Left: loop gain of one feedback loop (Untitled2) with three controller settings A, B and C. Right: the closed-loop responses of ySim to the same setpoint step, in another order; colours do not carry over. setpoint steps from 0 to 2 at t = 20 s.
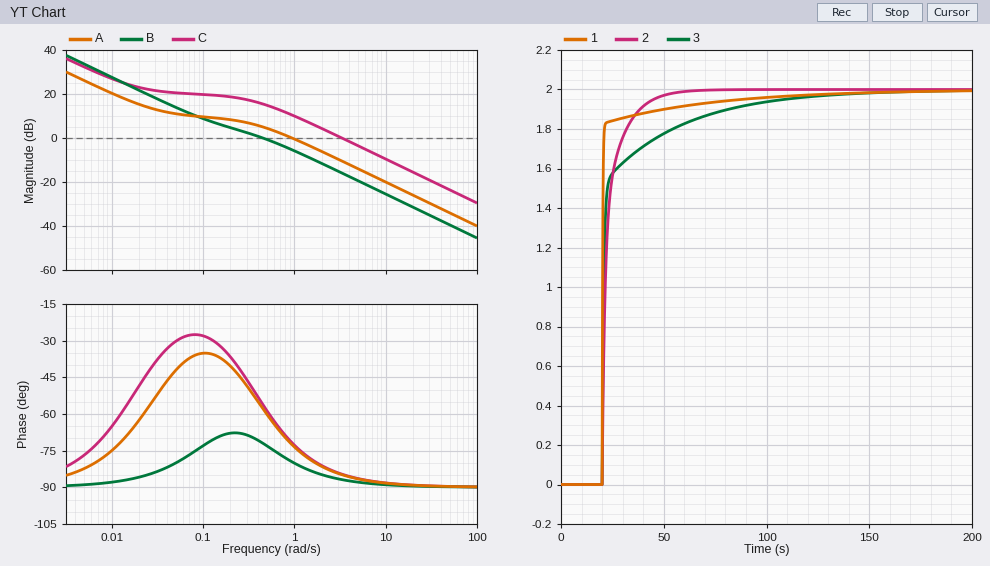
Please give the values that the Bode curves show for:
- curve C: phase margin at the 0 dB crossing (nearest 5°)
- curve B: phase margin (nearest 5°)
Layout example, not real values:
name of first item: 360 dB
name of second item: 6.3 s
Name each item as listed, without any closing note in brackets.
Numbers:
curve C: phase margin at the 0 dB crossing: 95°
curve B: phase margin: 110°
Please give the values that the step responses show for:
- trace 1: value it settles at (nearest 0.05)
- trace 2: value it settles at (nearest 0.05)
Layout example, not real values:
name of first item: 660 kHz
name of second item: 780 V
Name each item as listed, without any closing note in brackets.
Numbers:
trace 1: value it settles at: 2.00
trace 2: value it settles at: 2.00
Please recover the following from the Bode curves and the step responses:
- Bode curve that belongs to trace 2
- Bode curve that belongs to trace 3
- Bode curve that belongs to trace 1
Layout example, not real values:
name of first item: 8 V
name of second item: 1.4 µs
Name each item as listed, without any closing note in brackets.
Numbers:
Bode curve that belongs to trace 2: B
Bode curve that belongs to trace 3: A
Bode curve that belongs to trace 1: C
